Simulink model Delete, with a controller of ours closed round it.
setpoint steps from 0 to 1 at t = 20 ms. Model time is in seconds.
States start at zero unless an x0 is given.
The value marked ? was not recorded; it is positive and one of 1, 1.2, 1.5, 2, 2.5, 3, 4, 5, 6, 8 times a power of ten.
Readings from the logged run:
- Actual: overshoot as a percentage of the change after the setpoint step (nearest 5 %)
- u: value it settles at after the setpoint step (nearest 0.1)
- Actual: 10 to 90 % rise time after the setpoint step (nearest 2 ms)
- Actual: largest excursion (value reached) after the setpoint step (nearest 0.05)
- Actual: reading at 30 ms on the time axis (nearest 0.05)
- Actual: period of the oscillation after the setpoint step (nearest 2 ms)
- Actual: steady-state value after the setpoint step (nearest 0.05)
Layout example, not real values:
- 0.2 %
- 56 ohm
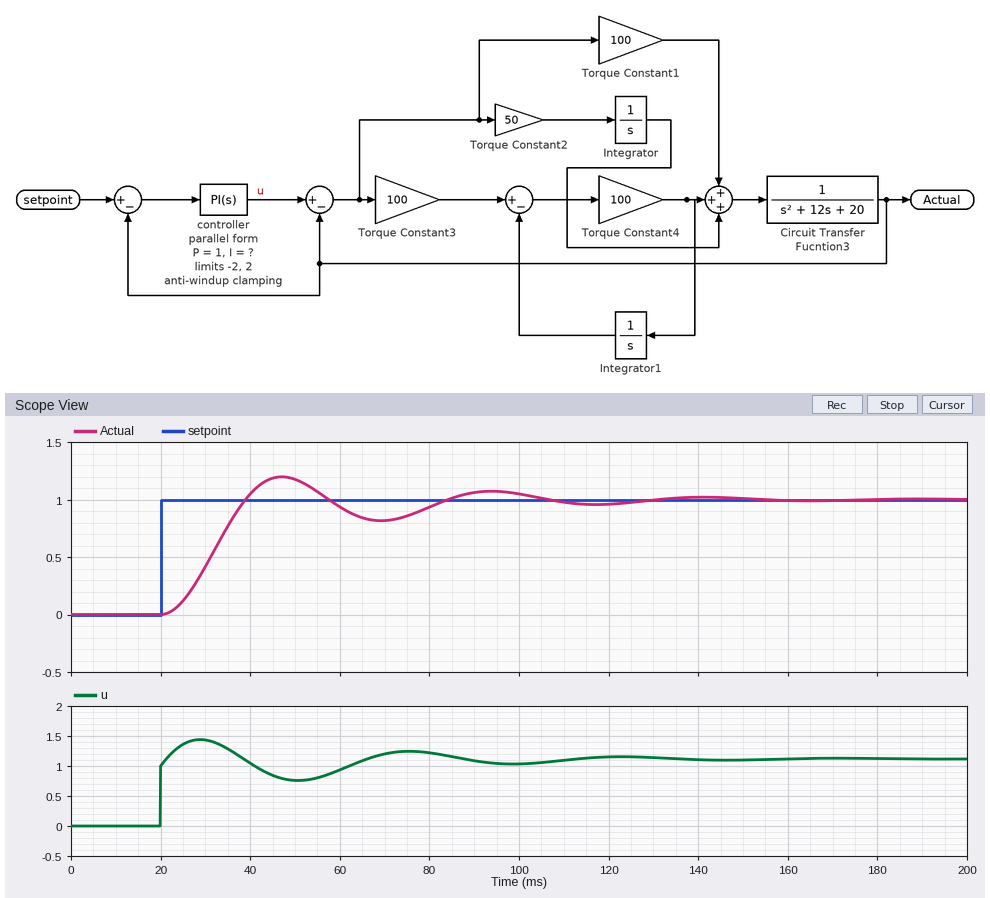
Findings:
- 20 %
- 1.1
- 12 ms
- 1.20
- 0.40
- 46 ms
- 1.00
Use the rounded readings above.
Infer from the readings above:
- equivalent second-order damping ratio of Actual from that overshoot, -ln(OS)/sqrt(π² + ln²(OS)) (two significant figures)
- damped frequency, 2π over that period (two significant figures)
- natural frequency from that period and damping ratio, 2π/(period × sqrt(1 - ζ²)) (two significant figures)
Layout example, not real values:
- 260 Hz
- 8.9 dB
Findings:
- 0.46
- 0.14 rad/ms
- 0.15 rad/ms
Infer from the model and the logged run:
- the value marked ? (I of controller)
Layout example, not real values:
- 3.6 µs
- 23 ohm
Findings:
- 100
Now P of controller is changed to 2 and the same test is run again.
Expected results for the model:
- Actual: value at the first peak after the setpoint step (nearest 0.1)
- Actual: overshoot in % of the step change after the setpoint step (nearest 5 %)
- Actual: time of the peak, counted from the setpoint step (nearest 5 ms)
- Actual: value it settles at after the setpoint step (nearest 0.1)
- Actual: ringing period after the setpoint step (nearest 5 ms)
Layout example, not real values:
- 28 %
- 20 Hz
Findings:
- 1.1
- 15 %
- 20 ms
- 1.0
- 40 ms
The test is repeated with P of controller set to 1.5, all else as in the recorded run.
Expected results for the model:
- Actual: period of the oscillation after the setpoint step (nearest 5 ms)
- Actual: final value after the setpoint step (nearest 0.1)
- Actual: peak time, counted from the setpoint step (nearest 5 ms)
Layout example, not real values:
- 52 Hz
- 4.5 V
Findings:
- 40 ms
- 1.0
- 25 ms
